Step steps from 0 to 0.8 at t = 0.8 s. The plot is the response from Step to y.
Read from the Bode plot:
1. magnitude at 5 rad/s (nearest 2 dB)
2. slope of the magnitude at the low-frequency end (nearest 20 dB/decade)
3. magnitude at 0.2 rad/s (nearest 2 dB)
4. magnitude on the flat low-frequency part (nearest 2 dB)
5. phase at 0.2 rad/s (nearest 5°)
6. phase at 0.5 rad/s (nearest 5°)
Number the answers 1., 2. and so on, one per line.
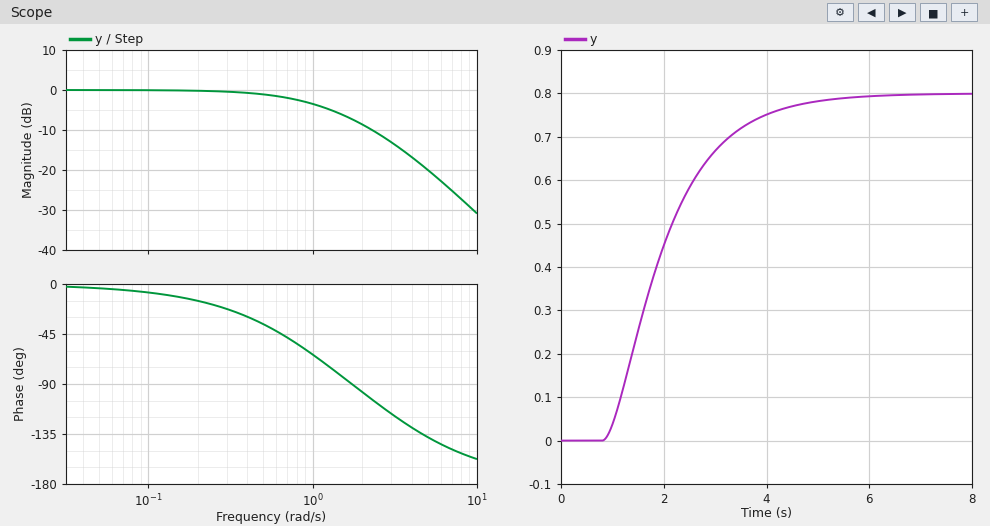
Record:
1. -20 dB
2. 0 dB/decade
3. 0 dB
4. 0 dB
5. -15°
6. -35°
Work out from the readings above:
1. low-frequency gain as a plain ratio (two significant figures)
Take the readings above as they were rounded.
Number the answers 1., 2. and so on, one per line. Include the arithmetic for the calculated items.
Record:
1. 10^(0 / 20) = 1.0
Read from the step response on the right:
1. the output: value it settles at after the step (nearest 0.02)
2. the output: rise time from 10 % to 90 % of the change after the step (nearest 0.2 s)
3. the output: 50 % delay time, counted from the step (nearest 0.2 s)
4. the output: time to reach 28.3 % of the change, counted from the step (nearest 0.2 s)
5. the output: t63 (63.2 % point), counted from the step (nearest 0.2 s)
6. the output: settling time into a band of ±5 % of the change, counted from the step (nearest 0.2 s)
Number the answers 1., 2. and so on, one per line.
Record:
1. 0.80
2. 2.4 s
3. 1.0 s
4. 0.6 s
5. 1.4 s
6. 3.4 s
